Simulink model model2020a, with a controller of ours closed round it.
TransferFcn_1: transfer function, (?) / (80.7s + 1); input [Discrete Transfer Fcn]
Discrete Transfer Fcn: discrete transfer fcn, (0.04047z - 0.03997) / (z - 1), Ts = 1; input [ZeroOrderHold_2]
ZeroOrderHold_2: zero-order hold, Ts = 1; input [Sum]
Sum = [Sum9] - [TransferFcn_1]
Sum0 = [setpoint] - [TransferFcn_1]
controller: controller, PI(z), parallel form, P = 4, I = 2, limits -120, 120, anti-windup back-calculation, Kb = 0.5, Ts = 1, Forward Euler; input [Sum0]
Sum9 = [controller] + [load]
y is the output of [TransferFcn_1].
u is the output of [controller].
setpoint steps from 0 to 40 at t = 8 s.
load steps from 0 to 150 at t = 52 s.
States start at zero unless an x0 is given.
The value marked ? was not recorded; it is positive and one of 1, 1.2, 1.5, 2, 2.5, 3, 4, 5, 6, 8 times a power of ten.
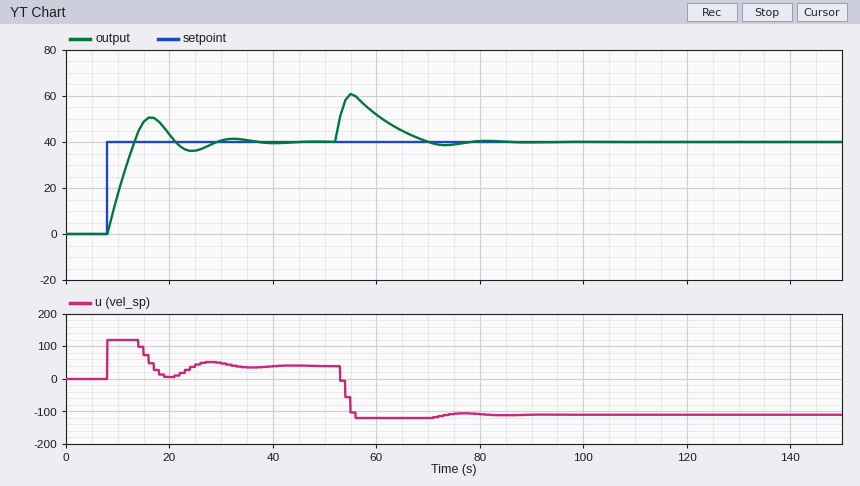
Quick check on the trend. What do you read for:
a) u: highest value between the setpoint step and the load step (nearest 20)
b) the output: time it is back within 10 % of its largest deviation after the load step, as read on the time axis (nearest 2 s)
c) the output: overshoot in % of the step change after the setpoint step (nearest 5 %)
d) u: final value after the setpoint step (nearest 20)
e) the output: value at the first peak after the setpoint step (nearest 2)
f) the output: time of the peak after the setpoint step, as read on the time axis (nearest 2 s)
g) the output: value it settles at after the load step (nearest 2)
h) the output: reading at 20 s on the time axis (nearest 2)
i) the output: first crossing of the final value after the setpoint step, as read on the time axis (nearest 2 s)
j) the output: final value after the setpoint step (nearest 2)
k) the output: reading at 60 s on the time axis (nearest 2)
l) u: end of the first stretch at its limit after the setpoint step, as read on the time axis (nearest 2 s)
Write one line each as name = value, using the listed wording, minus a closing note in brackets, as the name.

u: highest value between the setpoint step and the load step = 120
the output: time it is back within 10 % of its largest deviation after the load step, as read on the time axis = 68 s
the output: overshoot in % of the step change after the setpoint step = 25 %
u: final value after the setpoint step = 40
the output: value at the first peak after the setpoint step = 50
the output: time of the peak after the setpoint step, as read on the time axis = 16 s
the output: value it settles at after the load step = 40
the output: reading at 20 s on the time axis = 44
the output: first crossing of the final value after the setpoint step, as read on the time axis = 14 s
the output: final value after the setpoint step = 40
the output: reading at 60 s on the time axis = 52
u: end of the first stretch at its limit after the setpoint step, as read on the time axis = 14 s
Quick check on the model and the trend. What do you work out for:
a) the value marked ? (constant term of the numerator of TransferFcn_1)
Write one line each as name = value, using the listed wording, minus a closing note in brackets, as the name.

the value marked ? = 150
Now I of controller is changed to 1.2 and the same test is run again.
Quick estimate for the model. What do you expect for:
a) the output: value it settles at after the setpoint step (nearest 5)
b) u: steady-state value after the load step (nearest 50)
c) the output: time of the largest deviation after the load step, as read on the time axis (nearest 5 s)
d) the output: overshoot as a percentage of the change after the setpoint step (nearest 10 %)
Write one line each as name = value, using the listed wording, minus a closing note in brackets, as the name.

the output: value it settles at after the setpoint step = 40
u: steady-state value after the load step = -100
the output: time of the largest deviation after the load step, as read on the time axis = 55 s
the output: overshoot as a percentage of the change after the setpoint step = 20 %
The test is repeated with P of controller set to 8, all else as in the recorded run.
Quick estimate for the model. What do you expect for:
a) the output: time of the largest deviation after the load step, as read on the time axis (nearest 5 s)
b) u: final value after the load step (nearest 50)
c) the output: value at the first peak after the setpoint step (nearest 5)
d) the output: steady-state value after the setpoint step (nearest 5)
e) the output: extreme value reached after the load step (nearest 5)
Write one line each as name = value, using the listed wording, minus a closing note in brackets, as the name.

the output: time of the largest deviation after the load step, as read on the time axis = 55 s
u: final value after the load step = -100
the output: value at the first peak after the setpoint step = 40
the output: steady-state value after the setpoint step = 40
the output: extreme value reached after the load step = 55
